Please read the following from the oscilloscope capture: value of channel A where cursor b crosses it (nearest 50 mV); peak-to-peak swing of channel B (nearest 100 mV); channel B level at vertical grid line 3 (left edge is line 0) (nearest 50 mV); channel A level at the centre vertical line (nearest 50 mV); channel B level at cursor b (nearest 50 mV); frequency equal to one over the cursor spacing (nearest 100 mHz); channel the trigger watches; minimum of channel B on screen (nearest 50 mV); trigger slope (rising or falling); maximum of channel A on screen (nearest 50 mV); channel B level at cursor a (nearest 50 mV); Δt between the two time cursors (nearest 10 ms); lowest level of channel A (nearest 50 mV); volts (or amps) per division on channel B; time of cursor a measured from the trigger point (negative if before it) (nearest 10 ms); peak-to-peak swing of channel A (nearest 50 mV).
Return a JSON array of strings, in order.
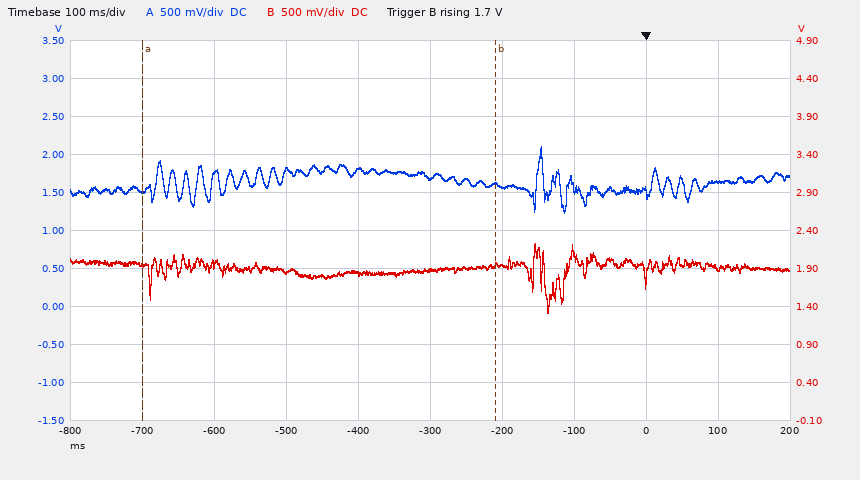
["1.60 V", "900 mV", "1.85 V", "1.70 V", "1.95 V", "2.0 Hz", "channel B", "1.30 V", "rising", "2.10 V", "1.95 V", "490 ms", "1.25 V", "500 mV", "-700 ms", "850 mV"]
